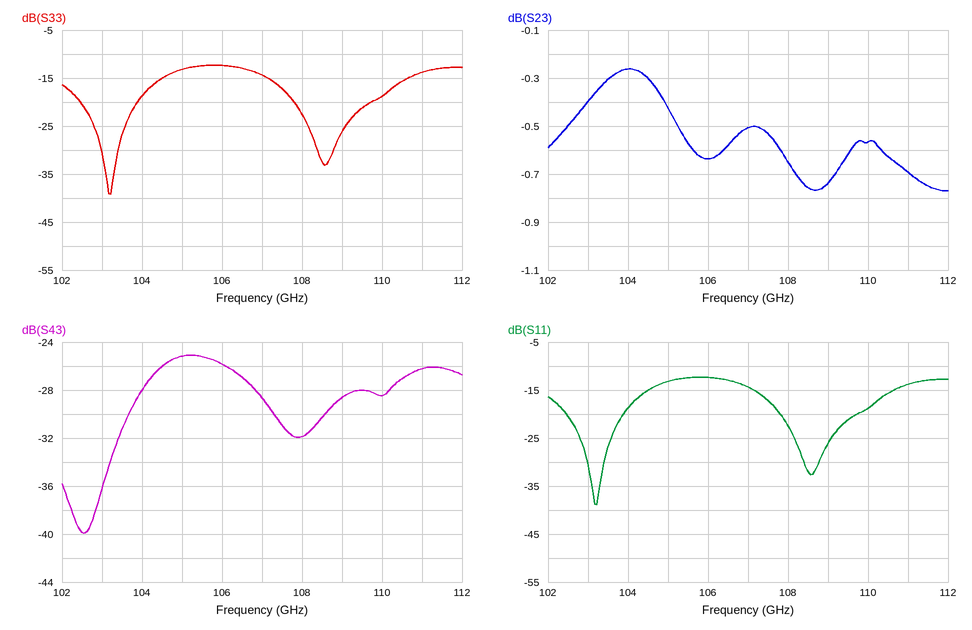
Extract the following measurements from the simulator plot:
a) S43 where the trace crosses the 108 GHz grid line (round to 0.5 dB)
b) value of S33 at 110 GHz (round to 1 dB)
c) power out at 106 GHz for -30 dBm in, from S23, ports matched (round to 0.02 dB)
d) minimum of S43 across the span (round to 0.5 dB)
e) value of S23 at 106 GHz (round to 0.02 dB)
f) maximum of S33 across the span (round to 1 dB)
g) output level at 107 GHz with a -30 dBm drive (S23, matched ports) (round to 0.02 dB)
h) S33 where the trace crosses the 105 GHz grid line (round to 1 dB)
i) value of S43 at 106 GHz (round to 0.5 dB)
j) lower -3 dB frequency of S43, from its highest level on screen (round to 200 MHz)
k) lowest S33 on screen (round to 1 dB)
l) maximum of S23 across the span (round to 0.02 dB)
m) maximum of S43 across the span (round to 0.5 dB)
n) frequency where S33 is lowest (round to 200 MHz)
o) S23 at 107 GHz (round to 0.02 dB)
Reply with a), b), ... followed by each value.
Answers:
a) -32.0 dB
b) -19 dB
c) -30.64 dBm
d) -40.0 dB
e) -0.64 dB
f) -12 dB
g) -30.50 dBm
h) -13 dB
i) -26.0 dB
j) 104.0 GHz
k) -39 dB
l) -0.26 dB
m) -25.0 dB
n) 103.2 GHz
o) -0.50 dB
